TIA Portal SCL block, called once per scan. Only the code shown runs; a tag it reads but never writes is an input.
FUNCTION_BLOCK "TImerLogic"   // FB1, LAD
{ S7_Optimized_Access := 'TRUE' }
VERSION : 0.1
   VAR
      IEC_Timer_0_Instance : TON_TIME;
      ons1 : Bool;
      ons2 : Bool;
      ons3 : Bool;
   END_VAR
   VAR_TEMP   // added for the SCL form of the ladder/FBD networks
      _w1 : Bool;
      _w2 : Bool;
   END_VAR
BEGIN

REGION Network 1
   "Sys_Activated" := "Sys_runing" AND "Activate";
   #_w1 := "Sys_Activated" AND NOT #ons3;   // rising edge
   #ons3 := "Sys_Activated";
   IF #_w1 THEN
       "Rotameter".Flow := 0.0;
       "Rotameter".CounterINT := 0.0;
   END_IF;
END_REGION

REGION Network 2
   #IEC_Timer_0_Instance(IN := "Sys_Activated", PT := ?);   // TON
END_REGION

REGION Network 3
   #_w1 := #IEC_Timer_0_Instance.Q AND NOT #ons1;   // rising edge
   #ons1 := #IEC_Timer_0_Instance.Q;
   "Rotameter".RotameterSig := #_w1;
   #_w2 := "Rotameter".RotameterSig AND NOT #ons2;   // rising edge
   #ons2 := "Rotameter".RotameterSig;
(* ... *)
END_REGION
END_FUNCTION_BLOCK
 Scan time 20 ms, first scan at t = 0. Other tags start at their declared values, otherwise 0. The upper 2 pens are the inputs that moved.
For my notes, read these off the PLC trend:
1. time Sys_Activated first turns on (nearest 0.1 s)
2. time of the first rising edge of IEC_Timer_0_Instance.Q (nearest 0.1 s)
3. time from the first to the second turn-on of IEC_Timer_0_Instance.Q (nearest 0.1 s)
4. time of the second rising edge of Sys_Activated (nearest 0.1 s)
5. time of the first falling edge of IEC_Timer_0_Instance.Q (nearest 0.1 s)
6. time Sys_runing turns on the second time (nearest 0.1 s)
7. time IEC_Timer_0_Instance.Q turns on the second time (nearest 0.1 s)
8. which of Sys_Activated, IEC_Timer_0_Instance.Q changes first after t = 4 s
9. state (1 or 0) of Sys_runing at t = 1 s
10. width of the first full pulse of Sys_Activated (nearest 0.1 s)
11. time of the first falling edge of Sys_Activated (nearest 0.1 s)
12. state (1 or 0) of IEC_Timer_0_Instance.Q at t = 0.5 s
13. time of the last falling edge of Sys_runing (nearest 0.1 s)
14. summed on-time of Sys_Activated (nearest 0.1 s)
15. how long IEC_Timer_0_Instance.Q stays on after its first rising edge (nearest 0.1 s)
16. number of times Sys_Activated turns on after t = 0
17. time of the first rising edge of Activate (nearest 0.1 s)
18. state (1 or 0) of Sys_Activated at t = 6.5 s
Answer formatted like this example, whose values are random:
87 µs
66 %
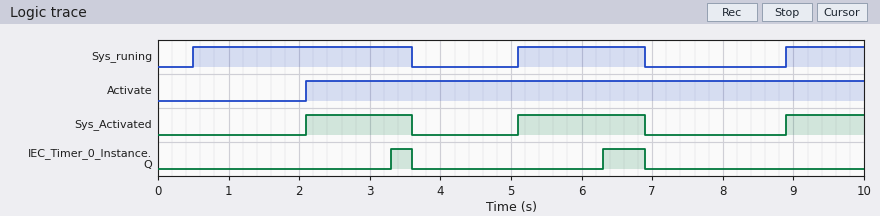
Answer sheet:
2.1 s
3.3 s
3.0 s
5.1 s
3.6 s
5.1 s
6.3 s
Sys_Activated
1
1.5 s
3.6 s
0
6.9 s
4.4 s
0.3 s
3
2.1 s
1
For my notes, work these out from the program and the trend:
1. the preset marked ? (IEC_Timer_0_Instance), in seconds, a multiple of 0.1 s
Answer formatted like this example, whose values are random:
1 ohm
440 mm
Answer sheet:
1.2 s
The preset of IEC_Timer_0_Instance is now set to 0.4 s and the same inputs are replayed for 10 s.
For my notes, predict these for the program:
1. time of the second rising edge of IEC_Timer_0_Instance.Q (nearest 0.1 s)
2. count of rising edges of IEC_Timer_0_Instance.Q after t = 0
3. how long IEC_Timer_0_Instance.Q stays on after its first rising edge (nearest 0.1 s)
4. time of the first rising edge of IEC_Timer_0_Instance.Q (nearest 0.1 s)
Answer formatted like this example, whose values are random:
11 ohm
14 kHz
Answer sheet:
5.5 s
3
1.1 s
2.5 s
